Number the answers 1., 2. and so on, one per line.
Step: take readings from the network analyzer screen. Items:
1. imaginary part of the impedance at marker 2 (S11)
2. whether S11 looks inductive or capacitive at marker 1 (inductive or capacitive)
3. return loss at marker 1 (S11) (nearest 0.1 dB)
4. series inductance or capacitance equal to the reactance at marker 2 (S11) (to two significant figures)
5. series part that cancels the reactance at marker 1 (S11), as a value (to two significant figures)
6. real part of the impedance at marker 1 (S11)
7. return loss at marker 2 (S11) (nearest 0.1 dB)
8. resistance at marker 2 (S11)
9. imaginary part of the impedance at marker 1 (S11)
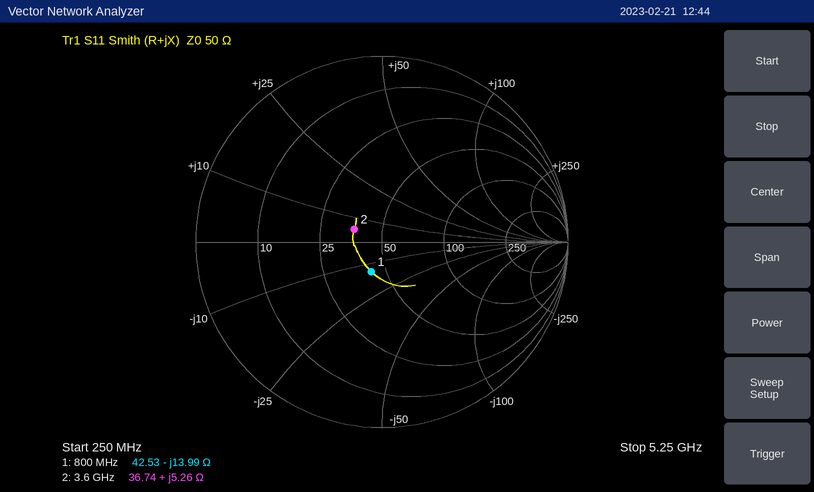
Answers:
1. +5.26 Ω
2. capacitive
3. 15.4 dB
4. 230 pH
5. 2.8 nH
6. 42.53 Ω
7. 15.7 dB
8. 36.74 Ω
9. -13.99 Ω
